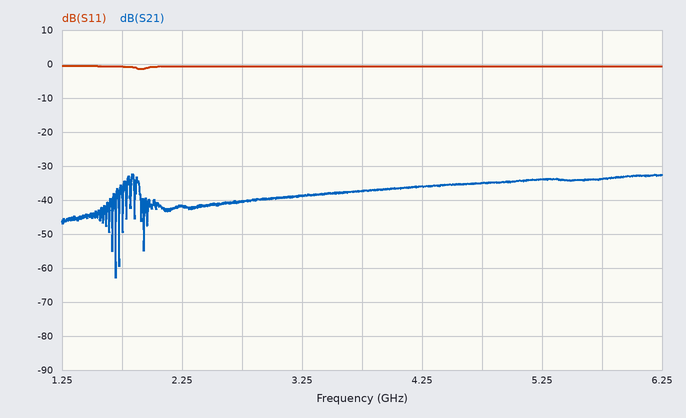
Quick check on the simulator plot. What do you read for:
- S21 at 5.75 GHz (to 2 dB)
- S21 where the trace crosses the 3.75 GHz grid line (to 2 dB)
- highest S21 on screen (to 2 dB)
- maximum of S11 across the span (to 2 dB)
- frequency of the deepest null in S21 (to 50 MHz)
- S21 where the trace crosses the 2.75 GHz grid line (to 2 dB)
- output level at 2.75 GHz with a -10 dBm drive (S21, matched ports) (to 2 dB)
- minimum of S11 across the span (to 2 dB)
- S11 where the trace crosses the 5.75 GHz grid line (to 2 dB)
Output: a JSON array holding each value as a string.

["-34 dB", "-38 dB", "-32 dB", "0 dB", "1.70 GHz", "-40 dB", "-50 dBm", "-2 dB", "0 dB"]
